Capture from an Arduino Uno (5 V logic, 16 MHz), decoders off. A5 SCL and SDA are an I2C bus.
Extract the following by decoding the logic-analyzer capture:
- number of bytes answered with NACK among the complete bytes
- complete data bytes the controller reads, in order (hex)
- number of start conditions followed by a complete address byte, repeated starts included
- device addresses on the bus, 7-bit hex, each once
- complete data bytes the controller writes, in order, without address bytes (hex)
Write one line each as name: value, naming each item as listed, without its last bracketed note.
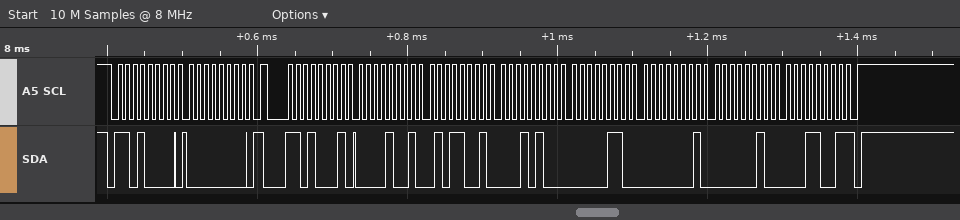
number of bytes answered with NACK among the complete bytes: 1
complete data bytes the controller reads, in order: 09 59 14 06 01 02 19
number of start conditions followed by a complete address byte, repeated starts included: 2
device addresses on the bus, 7-bit hex, each once: 0x68
complete data bytes the controller writes, in order, without address bytes: 00
